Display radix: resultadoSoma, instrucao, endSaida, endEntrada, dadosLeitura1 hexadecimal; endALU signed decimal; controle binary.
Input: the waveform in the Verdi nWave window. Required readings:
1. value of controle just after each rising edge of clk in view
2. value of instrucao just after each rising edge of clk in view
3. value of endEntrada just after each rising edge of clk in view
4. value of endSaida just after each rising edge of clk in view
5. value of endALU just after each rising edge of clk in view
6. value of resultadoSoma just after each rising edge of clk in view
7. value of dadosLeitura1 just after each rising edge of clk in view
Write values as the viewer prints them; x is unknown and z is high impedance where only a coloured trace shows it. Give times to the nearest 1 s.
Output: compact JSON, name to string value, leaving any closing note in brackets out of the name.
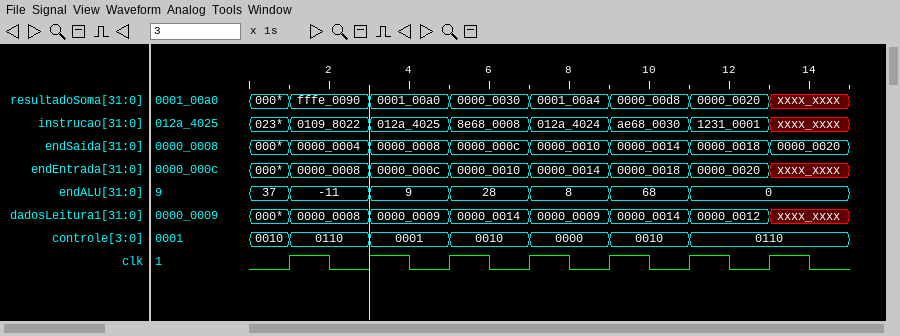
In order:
{"value of controle just after each rising edge of clk in view": "0110, 0001, 0010, 0000, 0010, 0110, 0110", "value of instrucao just after each rising edge of clk in view": "0109_8022, 012a_4025, 8e68_0008, 012a_4024, ae68_0030, 1231_0001, xxxx_xxxx", "value of endEntrada just after each rising edge of clk in view": "0000_0008, 0000_000c, 0000_0010, 0000_0014, 0000_0018, 0000_0020, xxxx_xxxx", "value of endSaida just after each rising edge of clk in view": "0000_0004, 0000_0008, 0000_000c, 0000_0010, 0000_0014, 0000_0018, 0000_0020", "value of endALU just after each rising edge of clk in view": "-11, 9, 28, 8, 68, 0, 0", "value of resultadoSoma just after each rising edge of clk in view": "fffe_0090, 0001_00a0, 0000_0030, 0001_00a4, 0000_00d8, 0000_0020, xxxx_xxxx", "value of dadosLeitura1 just after each rising edge of clk in view": "0000_0008, 0000_0009, 0000_0014, 0000_0009, 0000_0014, 0000_0012, xxxx_xxxx"}
